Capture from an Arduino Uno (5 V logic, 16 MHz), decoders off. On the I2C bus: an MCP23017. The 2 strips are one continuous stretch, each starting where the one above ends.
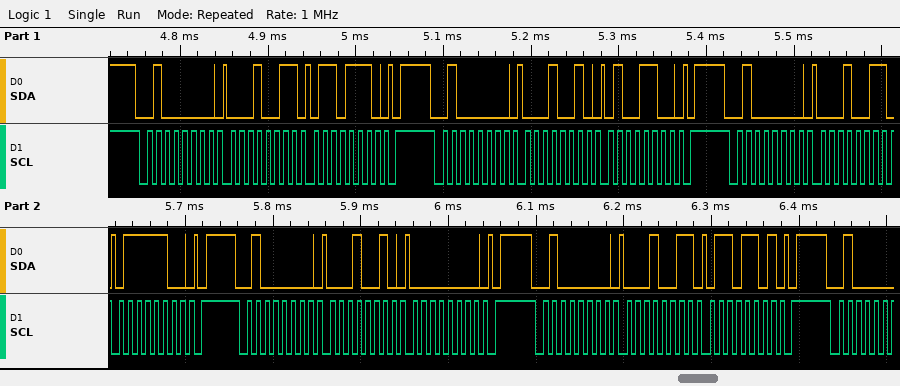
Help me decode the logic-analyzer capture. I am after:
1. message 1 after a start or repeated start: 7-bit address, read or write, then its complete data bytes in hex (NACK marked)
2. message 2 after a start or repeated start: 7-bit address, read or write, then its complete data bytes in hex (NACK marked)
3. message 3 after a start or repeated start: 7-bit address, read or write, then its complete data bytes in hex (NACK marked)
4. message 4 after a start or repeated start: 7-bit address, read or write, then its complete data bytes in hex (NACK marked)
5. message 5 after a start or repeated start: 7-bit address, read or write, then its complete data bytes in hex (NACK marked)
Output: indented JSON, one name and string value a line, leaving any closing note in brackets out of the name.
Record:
{
  "message 1 after a start or repeated start: 7-bit address, read or write, then its complete data bytes in hex": "0x20 write: 13 6E",
  "message 2 after a start or repeated start: 7-bit address, read or write, then its complete data bytes in hex": "0x20 write: 12 4C",
  "message 3 after a start or repeated start: 7-bit address, read or write, then its complete data bytes in hex": "0x20 write: 13 7C",
  "message 4 after a start or repeated start: 7-bit address, read or write, then its complete data bytes in hex": "0x20 write: 12 00",
  "message 5 after a start or repeated start: 7-bit address, read or write, then its complete data bytes in hex": "0x20 write: 13 6D"
}
